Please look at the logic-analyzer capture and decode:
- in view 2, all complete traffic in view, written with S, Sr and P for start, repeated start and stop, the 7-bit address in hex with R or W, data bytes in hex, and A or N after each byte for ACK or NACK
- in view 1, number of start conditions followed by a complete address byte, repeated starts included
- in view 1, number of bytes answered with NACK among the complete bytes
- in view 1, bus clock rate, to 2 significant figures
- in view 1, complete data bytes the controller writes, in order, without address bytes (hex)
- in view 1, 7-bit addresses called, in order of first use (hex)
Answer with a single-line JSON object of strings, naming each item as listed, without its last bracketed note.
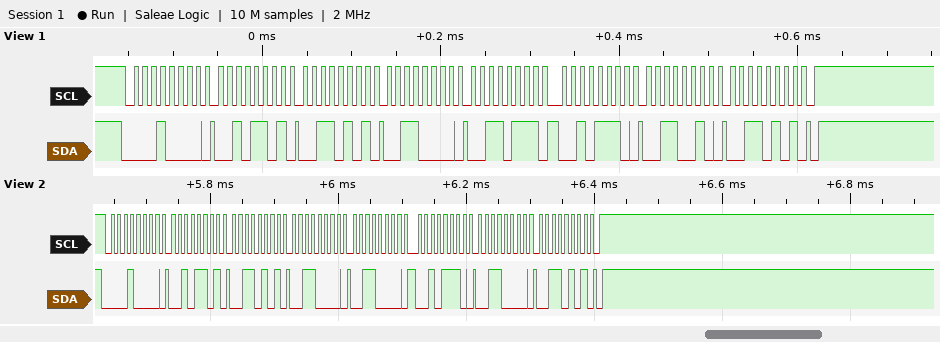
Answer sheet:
{"in view 2, all complete traffic in view, written with S, Sr and P for start, repeated start and stop, the 7-bit address in hex with R or W, data bytes in hex, and A or N after each byte for ACK or NACK": "S 08W A 2D A 35 A 30 A 30 A 2E A 30 A 35 A P", "in view 1, number of start conditions followed by a complete address byte, repeated starts included": "1", "in view 1, number of bytes answered with NACK among the complete bytes": "0", "in view 1, bus clock rate, to 2 significant figures": "100 kHz", "in view 1, complete data bytes the controller writes, in order, without address bytes": "2D 35 30 37 2E 32 35", "in view 1, 7-bit addresses called, in order of first use": "0x08"}
